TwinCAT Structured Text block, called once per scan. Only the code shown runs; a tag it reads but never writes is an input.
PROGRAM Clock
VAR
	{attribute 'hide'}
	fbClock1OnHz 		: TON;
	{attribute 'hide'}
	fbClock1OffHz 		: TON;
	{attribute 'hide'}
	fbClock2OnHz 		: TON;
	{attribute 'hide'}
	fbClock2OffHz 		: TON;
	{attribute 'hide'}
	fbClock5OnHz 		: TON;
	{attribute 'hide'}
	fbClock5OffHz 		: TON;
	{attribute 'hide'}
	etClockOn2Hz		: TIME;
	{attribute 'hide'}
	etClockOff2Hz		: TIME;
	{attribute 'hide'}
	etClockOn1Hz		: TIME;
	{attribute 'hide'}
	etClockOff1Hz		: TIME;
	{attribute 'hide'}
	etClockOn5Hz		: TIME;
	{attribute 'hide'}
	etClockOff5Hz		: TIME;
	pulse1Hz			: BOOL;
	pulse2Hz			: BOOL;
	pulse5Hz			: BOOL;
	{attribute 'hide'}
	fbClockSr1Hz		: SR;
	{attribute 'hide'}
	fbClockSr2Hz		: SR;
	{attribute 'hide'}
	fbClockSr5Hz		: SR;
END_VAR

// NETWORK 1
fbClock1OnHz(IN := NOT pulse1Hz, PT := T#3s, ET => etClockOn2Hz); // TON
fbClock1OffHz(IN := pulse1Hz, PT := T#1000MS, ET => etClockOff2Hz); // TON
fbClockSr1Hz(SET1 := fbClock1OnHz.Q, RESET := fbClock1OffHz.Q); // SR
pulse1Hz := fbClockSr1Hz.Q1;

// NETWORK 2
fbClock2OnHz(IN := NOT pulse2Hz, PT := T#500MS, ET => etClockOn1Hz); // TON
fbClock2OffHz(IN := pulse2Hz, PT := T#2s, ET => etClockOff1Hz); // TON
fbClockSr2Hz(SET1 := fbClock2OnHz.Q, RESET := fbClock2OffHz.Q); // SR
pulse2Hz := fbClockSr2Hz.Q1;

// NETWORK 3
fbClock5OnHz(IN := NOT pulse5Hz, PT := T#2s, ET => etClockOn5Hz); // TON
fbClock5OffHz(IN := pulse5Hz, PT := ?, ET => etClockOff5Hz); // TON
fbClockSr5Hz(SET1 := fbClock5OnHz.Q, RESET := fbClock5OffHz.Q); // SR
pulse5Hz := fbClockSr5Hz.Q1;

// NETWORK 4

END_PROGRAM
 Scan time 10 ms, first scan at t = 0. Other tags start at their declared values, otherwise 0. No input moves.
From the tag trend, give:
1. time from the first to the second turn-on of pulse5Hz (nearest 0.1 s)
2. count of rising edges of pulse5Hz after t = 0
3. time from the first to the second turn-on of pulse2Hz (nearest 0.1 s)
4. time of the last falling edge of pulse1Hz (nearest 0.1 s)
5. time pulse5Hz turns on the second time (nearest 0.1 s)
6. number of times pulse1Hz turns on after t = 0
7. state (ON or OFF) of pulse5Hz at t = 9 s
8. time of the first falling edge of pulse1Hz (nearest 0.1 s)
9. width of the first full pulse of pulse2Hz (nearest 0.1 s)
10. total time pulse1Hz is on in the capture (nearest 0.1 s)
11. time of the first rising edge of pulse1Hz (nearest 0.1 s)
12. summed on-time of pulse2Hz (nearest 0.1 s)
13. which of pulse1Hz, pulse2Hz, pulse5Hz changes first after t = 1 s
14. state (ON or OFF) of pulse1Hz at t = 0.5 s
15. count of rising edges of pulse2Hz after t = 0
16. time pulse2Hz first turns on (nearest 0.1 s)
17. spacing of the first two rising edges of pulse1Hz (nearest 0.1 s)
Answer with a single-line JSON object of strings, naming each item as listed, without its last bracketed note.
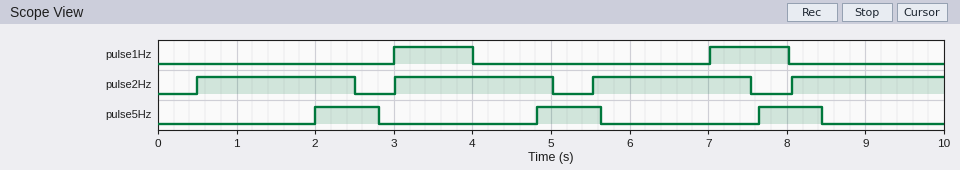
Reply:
{"time from the first to the second turn-on of pulse5Hz": "2.8 s", "count of rising edges of pulse5Hz after t = 0": "3", "time from the first to the second turn-on of pulse2Hz": "2.5 s", "time of the last falling edge of pulse1Hz": "8.0 s", "time pulse5Hz turns on the second time": "4.8 s", "number of times pulse1Hz turns on after t = 0": "2", "state (ON or OFF) of pulse5Hz at t = 9 s": "OFF", "time of the first falling edge of pulse1Hz": "4.0 s", "width of the first full pulse of pulse2Hz": "2.0 s", "total time pulse1Hz is on in the capture": "2.0 s", "time of the first rising edge of pulse1Hz": "3.0 s", "summed on-time of pulse2Hz": "8.0 s", "which of pulse1Hz, pulse2Hz, pulse5Hz changes first after t = 1 s": "pulse5Hz", "state (ON or OFF) of pulse1Hz at t = 0.5 s": "OFF", "count of rising edges of pulse2Hz after t = 0": "4", "time pulse2Hz first turns on": "0.5 s", "spacing of the first two rising edges of pulse1Hz": "4.0 s"}
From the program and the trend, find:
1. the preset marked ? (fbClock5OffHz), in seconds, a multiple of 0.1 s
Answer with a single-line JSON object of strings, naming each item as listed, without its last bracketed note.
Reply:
{"the preset marked ? (fbClock5OffHz), in seconds, a multiple of 0.1 s": "0.8 s"}
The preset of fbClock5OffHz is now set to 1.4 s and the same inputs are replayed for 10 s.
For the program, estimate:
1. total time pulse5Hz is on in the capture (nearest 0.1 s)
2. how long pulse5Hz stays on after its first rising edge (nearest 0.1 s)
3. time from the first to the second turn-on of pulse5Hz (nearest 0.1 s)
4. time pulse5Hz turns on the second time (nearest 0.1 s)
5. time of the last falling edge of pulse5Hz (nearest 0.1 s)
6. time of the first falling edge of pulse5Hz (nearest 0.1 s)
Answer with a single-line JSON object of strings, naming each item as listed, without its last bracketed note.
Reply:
{"total time pulse5Hz is on in the capture": "4.0 s", "how long pulse5Hz stays on after its first rising edge": "1.4 s", "time from the first to the second turn-on of pulse5Hz": "3.4 s", "time pulse5Hz turns on the second time": "5.4 s", "time of the last falling edge of pulse5Hz": "6.8 s", "time of the first falling edge of pulse5Hz": "3.4 s"}
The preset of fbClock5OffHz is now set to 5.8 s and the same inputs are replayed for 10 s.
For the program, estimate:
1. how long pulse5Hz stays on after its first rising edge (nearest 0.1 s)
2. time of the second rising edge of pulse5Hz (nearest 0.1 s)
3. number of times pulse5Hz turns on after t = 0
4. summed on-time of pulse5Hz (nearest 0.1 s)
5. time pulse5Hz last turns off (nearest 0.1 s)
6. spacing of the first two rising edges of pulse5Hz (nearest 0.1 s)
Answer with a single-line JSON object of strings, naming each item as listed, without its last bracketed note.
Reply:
{"how long pulse5Hz stays on after its first rising edge": "5.8 s", "time of the second rising edge of pulse5Hz": "9.8 s", "number of times pulse5Hz turns on after t = 0": "2", "summed on-time of pulse5Hz": "6.0 s", "time pulse5Hz last turns off": "7.8 s", "spacing of the first two rising edges of pulse5Hz": "7.8 s"}
